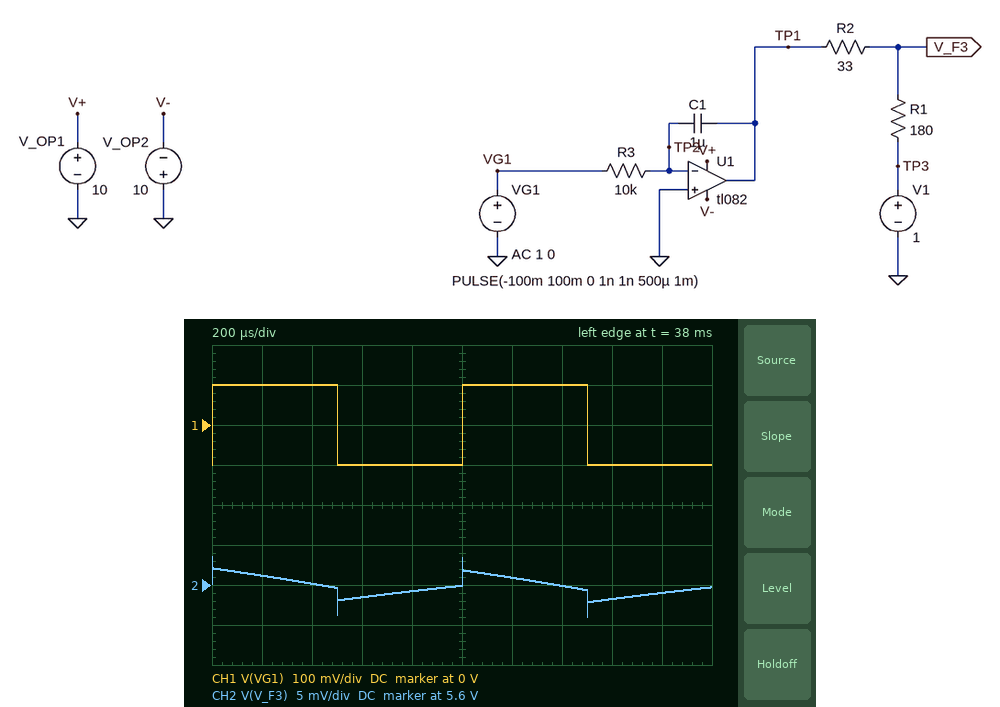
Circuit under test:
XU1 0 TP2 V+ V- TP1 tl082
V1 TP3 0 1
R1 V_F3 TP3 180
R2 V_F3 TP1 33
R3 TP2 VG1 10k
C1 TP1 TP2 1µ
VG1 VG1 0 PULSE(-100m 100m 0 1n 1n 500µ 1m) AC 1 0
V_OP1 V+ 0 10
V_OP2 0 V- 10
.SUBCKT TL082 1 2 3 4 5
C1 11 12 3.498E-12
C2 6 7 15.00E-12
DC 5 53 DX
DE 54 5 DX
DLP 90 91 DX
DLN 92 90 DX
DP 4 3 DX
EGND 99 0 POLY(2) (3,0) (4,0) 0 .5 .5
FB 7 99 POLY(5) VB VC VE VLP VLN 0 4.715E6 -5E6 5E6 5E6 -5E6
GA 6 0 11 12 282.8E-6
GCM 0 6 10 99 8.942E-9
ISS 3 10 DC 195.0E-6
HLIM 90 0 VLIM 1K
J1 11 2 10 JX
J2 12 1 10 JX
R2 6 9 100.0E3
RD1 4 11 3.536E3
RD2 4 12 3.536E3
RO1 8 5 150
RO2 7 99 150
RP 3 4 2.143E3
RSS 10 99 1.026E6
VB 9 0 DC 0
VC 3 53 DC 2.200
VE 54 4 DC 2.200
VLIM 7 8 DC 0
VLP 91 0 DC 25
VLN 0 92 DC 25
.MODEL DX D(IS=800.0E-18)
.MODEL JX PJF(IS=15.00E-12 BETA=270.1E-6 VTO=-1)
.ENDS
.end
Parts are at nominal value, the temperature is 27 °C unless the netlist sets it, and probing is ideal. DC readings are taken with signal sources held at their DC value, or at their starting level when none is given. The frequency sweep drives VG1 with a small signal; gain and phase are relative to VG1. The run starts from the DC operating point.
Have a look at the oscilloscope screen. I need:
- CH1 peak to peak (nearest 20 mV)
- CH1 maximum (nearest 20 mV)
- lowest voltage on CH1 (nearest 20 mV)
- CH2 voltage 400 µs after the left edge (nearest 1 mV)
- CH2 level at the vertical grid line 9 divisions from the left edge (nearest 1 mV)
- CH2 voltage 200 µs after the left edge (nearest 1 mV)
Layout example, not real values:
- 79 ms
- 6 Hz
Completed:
- 200 mV
- 100 mV
- -100 mV
- 5.600 V
- 5.599 V
- 5.601 V
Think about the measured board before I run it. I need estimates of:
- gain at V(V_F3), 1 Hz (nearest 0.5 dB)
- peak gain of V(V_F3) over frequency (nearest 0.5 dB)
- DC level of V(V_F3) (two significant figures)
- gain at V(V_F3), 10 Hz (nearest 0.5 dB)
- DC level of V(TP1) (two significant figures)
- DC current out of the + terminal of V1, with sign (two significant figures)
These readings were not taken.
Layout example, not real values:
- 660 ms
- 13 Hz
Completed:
- -26.5 dB
- -26.5 dB
- 5.6 V
- -28.0 dB
- 6.5 V
- -26 mA
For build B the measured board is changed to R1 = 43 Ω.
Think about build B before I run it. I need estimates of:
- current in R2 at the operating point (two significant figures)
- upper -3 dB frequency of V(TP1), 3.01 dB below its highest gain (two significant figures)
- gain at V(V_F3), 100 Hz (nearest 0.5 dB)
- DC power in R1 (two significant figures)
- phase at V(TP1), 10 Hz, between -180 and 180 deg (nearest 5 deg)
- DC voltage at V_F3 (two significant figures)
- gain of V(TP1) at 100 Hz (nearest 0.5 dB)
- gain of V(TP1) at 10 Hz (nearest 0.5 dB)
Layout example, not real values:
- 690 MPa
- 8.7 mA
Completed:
- 26 mA
- 18 Hz
- -47.0 dB
- 28 mW
- 135 deg
- 2.1 V
- -42.0 dB
- -35.5 dB
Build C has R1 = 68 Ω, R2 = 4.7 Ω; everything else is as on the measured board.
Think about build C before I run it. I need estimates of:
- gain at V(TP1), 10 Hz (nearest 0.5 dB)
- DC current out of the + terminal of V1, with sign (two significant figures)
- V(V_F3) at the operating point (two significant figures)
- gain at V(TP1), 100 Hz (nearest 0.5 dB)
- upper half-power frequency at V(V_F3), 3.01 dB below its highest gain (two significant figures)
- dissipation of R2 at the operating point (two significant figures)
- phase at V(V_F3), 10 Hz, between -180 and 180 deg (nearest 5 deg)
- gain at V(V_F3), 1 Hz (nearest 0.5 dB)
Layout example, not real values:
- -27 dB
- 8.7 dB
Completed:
- -36.0 dB
- -26 mA
- 2.7 V
- -42.5 dB
- 18 Hz
- 3.1 mW
- 135 deg
- -35.0 dB
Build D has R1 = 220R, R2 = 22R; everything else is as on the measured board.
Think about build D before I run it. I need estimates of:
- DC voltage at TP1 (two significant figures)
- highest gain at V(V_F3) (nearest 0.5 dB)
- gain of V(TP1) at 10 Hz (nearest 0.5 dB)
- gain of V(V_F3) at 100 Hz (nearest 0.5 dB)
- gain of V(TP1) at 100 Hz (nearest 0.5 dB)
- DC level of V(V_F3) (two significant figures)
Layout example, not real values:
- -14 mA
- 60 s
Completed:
- 7.2 V
- -25.0 dB
- -25.5 dB
- -33.5 dB
- -32.5 dB
- 6.6 V
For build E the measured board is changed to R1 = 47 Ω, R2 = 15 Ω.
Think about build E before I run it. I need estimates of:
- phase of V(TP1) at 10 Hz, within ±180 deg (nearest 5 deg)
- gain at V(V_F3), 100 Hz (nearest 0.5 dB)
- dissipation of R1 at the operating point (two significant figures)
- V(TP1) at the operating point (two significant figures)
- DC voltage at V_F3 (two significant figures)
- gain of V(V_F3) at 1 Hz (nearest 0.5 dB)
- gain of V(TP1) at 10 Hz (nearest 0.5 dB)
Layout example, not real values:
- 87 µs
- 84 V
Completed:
- 135 deg
- -46.0 dB
- 31 mW
- 2.6 V
- 2.2 V
- -38.5 dB
- -37.0 dB
